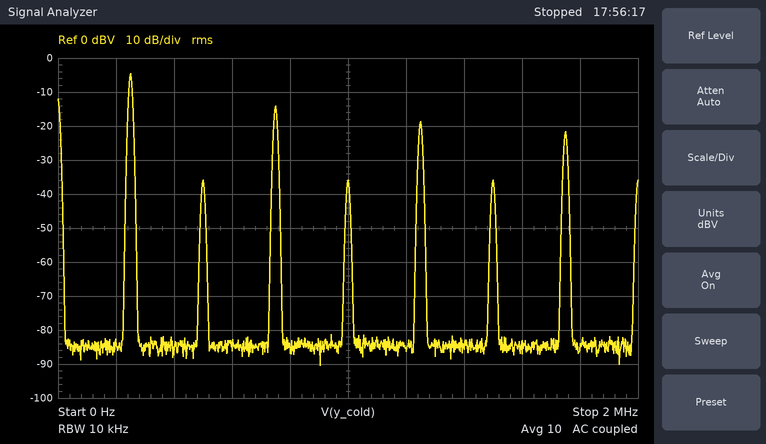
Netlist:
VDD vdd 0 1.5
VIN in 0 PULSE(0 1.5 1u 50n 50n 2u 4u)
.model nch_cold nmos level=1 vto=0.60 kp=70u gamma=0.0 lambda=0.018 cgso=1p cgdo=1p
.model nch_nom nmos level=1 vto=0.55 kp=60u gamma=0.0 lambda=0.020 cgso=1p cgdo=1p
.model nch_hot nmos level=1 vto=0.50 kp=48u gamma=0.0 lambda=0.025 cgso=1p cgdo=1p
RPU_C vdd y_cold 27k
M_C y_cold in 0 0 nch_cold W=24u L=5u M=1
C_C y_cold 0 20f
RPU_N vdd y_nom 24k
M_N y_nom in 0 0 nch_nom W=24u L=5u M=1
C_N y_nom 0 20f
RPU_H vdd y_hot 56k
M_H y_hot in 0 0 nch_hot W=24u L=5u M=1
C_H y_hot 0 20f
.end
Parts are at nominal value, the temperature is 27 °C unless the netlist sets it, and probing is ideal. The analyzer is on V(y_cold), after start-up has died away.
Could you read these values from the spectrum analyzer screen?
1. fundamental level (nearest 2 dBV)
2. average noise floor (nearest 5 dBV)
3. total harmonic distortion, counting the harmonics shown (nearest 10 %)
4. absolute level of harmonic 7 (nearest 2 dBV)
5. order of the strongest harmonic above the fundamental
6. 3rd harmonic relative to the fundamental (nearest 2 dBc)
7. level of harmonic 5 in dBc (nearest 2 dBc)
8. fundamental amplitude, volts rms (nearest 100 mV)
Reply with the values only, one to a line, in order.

-4 dBV
-85 dBV
40 %
-22 dBV
3
-10 dBc
-14 dBc
600 mV
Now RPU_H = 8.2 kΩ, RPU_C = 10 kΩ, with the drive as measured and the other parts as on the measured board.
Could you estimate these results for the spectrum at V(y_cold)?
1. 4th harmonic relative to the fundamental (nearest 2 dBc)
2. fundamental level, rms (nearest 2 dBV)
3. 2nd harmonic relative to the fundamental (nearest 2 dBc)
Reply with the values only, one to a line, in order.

-34 dBc
-6 dBV
-34 dBc
